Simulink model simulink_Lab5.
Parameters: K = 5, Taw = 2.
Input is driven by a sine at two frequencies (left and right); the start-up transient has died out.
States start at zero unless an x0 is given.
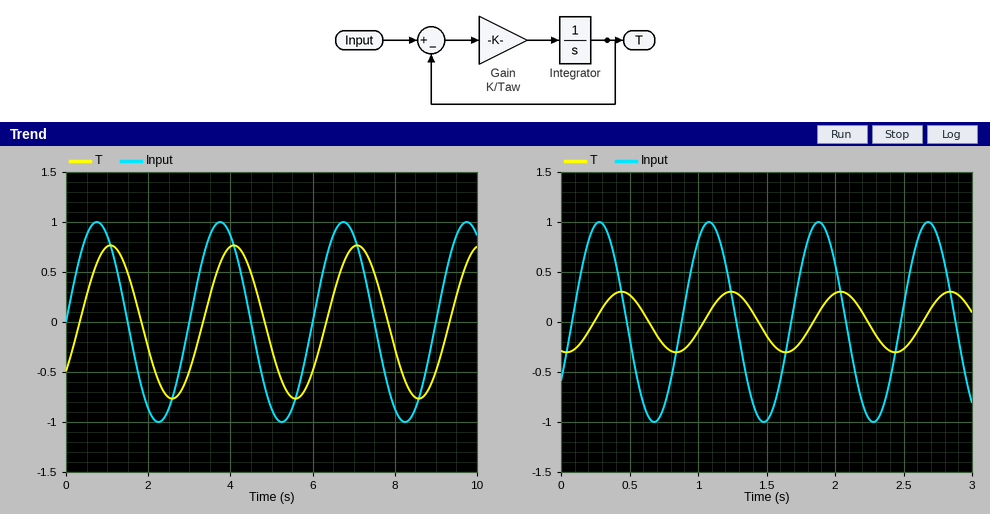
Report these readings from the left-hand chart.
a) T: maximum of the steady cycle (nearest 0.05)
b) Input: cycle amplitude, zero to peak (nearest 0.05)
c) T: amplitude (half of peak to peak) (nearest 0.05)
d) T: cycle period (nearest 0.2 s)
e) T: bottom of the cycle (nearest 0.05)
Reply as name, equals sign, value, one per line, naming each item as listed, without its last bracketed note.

T: maximum of the steady cycle = 0.75
Input: cycle amplitude, zero to peak = 1.00
T: amplitude (half of peak to peak) = 0.75
T: cycle period = 3.0 s
T: bottom of the cycle = -0.75
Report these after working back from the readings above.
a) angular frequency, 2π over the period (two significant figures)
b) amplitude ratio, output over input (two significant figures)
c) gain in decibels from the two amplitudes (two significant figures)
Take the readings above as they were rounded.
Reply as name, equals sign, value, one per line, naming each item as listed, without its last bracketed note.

angular frequency, 2π over the period = 2.1 rad/s
amplitude ratio, output over input = 0.75
gain in decibels from the two amplitudes = -2.5 dB
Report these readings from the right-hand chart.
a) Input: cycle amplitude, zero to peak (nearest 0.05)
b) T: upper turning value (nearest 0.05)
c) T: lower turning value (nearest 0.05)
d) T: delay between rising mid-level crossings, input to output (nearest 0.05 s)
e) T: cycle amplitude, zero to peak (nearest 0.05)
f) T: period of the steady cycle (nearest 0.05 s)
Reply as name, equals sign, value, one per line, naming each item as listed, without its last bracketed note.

Input: cycle amplitude, zero to peak = 1.00
T: upper turning value = 0.30
T: lower turning value = -0.30
T: delay between rising mid-level crossings, input to output = 0.15 s
T: cycle amplitude, zero to peak = 0.30
T: period of the steady cycle = 0.80 s
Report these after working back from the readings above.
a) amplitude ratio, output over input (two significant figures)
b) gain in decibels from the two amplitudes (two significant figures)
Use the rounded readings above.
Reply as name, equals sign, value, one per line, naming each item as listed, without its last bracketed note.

amplitude ratio, output over input = 0.30
gain in decibels from the two amplitudes = -10 dB
